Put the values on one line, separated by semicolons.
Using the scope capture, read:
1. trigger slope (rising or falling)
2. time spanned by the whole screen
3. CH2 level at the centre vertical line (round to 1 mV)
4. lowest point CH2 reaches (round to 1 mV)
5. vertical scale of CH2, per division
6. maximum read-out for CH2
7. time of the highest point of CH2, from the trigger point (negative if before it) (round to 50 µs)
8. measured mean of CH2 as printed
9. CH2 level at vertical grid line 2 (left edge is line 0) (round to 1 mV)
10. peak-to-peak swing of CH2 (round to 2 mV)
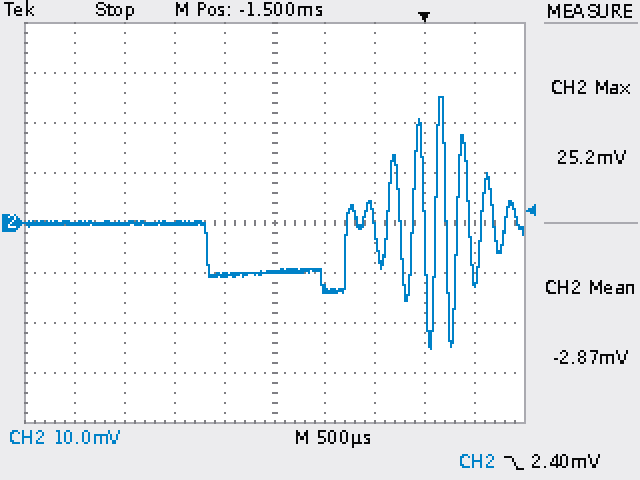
falling; 5 ms; -10 mV; -25 mV; 10 mV; 25.2 mV; +150 µs; -2.87 mV; 0 mV; 50 mV
